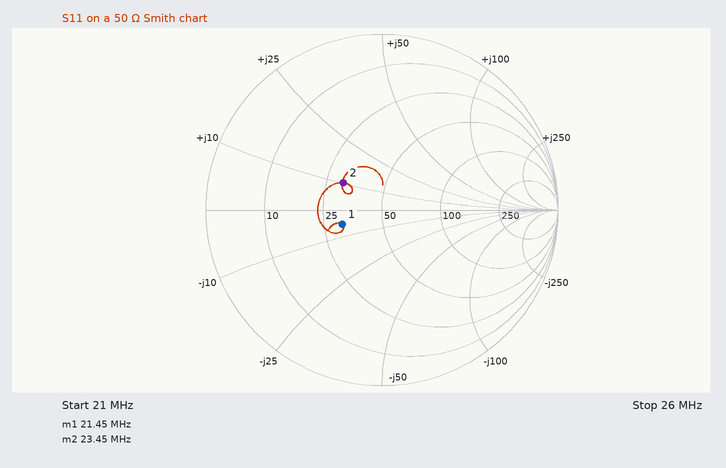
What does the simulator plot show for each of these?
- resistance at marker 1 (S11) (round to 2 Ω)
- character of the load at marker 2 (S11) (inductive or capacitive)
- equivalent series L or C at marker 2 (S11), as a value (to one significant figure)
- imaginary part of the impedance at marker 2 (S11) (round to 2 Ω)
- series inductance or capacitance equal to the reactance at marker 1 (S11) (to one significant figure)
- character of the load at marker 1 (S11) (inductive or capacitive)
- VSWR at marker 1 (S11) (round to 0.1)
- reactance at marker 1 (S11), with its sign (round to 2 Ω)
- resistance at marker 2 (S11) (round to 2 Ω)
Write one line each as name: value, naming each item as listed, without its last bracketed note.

resistance at marker 1 (S11): 32 Ω
character of the load at marker 2 (S11): inductive
equivalent series L or C at marker 2 (S11), as a value: 70 nH
imaginary part of the impedance at marker 2 (S11): +10 Ω
series inductance or capacitance equal to the reactance at marker 1 (S11): 1 nF
character of the load at marker 1 (S11): capacitive
VSWR at marker 1 (S11): 1.6
reactance at marker 1 (S11), with its sign: -6 Ω
resistance at marker 2 (S11): 30 Ω
